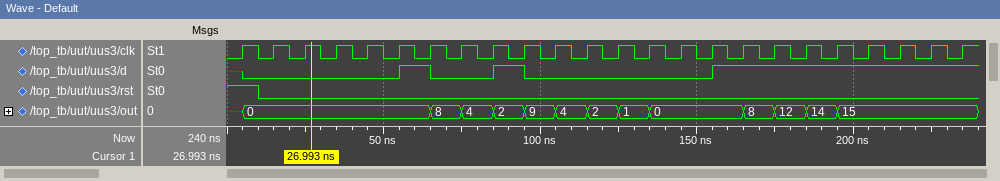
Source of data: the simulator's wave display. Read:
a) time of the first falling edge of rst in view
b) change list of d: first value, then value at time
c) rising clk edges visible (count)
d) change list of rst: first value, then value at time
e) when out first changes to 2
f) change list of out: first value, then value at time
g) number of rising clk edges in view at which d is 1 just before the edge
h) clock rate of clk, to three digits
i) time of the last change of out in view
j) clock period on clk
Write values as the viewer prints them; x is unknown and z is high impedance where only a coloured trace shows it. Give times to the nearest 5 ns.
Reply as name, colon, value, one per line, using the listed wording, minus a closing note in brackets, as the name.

time of the first falling edge of rst in view: 10 ns
change list of d: first value, then value at time: x, 0 at 5 ns, 1 at 55 ns, 0 at 65 ns, 1 at 85 ns, 0 at 95 ns, 1 at 155 ns
rising clk edges visible: 24
change list of rst: first value, then value at time: 1, 0 at 10 ns
when out first changes to 2: 85 ns
change list of out: first value, then value at time: x, 0 at 5 ns, 8 at 65 ns, 4 at 75 ns, 2 at 85 ns, 9 at 95 ns, 4 at 105 ns, 2 at 115 ns, 1 at 125 ns, 0 at 135 ns, 8 at 165 ns, 12 at 175 ns, 14 at 185 ns, 15 at 195 ns
number of rising clk edges in view at which d is 1 just before the edge: 10
clock rate of clk, to three digits: 100 MHz
time of the last change of out in view: 195 ns
clock period on clk: 10 ns
